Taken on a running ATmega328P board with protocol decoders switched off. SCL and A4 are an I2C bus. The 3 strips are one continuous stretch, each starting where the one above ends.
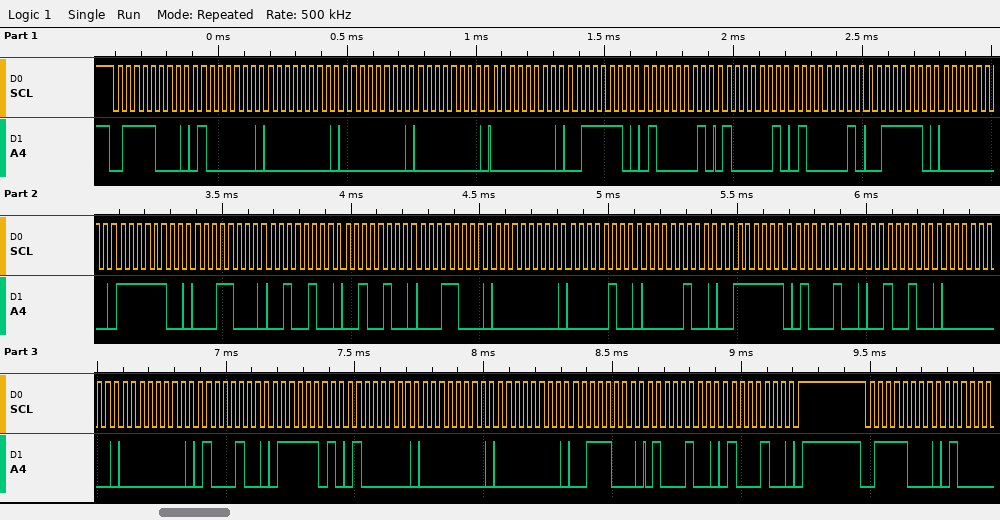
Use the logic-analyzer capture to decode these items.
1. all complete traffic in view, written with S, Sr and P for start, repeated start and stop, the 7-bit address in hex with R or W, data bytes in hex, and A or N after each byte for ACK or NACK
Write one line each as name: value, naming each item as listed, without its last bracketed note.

all complete traffic in view, written with S, Sr and P for start, repeated start and stop, the 7-bit address in hex with R or W, data bytes in hex, and A or N after each byte for ACK or NACK: S 3CW A 40 A 00 A 00 A 00 A 00 A 3E A 41 A 41 A 41 A 3E A 00 A FC A 18 A 24 A 24 A 18 A 00 A 04 A 04 A 3F A 44 A 24 A 00 A 00 A 44 A 7D A 40 A 00 A 00 A 38 A 44 A 44 A P S 3CW A
